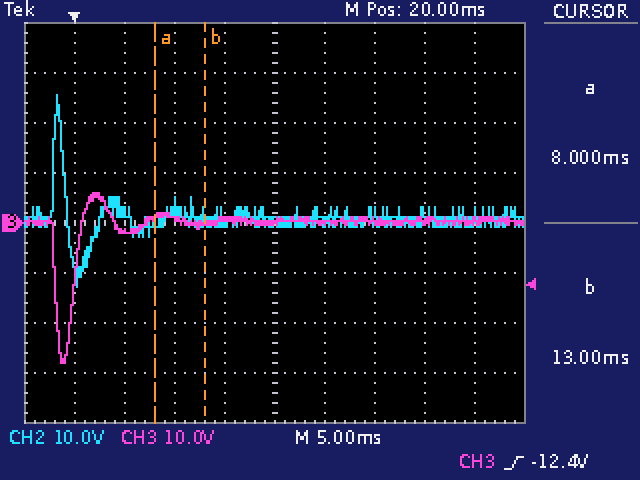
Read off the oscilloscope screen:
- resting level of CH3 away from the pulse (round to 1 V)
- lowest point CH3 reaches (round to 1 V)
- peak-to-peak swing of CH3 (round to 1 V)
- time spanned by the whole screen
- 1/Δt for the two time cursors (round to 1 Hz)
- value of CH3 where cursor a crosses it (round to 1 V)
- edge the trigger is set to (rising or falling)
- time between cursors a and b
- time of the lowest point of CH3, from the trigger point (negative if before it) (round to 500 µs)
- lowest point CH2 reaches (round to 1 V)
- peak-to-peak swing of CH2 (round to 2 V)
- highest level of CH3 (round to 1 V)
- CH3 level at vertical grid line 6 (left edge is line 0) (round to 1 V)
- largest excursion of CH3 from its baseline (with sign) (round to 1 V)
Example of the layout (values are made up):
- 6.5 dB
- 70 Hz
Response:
- 0 V
- -28 V
- 34 V
- 50 ms
- 200 Hz
- 1 V
- rising
- 5.0 ms
- -1.0 ms
- -13 V
- 38 V
- 6 V
- 0 V
- -28 V
